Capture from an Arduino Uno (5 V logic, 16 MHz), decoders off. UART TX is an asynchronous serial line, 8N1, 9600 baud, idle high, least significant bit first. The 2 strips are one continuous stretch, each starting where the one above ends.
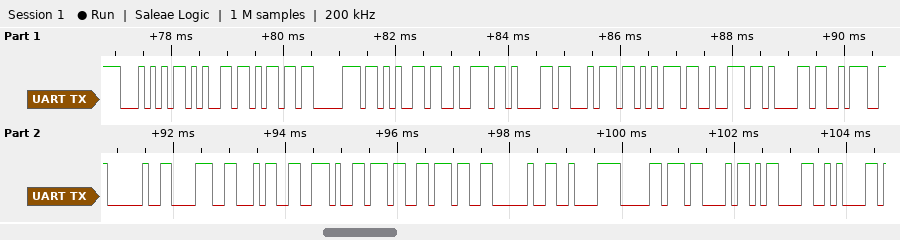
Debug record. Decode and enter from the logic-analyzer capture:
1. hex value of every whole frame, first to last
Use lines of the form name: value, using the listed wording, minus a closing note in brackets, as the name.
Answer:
hex value of every whole frame, first to last: 54 65 6D 70 65 72 61 74 75 72 61 3A 20 38 34 2E 37 37 20 C2 B0 43 0D 0A
